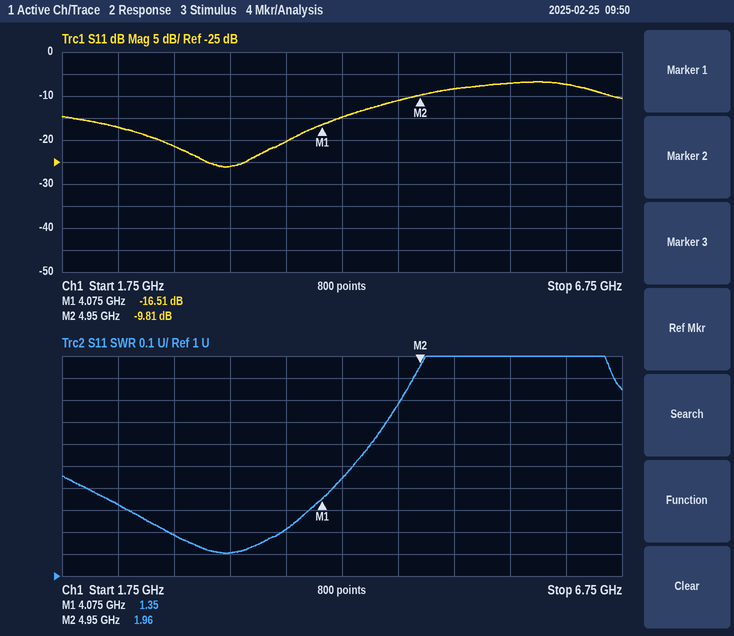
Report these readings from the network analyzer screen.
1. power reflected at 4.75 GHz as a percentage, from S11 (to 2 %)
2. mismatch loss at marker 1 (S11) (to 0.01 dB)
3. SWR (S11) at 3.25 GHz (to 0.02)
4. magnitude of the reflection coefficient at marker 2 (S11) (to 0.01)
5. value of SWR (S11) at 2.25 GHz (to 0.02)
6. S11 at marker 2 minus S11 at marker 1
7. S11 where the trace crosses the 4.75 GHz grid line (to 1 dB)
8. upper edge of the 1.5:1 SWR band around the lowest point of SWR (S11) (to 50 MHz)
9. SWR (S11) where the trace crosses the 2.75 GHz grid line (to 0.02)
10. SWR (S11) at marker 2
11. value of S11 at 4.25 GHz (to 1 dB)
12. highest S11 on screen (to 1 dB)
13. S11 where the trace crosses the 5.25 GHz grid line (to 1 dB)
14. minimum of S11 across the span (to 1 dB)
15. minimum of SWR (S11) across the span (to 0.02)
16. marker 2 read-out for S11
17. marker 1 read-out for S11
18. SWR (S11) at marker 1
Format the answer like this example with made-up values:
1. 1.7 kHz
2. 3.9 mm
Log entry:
1. 8 %
2. 0.10 dB
3. 1.10
4. 0.32
5. 1.32
6. 6.70 dB
7. -11 dB
8. 4.35 GHz
9. 1.18
10. 1.96
11. -15 dB
12. -7 dB
13. -8 dB
14. -26 dB
15. 1.10
16. -9.81 dB
17. -16.51 dB
18. 1.35
